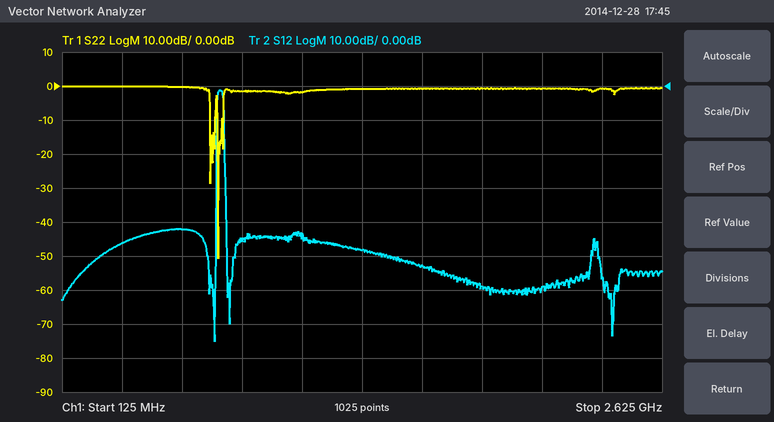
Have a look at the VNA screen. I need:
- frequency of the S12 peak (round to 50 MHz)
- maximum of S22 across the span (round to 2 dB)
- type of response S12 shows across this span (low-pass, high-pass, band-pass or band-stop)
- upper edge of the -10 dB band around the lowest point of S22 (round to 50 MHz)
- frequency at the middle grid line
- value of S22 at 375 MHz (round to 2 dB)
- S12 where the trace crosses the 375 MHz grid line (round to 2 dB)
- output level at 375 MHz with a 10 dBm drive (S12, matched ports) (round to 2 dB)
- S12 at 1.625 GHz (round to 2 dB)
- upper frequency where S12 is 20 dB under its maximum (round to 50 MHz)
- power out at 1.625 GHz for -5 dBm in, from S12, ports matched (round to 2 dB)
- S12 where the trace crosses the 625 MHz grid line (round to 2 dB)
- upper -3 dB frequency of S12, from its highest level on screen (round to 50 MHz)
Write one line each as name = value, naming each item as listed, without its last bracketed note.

frequency of the S12 peak = 800 MHz
maximum of S22 across the span = 0 dB
type of response S12 shows across this span = band-pass
upper edge of the -10 dB band around the lowest point of S22 = 800 MHz
frequency at the middle grid line = 1.375 GHz
value of S22 at 375 MHz = 0 dB
S12 where the trace crosses the 375 MHz grid line = -46 dB
output level at 375 MHz with a 10 dBm drive (S12, matched ports) = -36 dBm
S12 at 1.625 GHz = -52 dB
upper frequency where S12 is 20 dB under its maximum = 800 MHz
power out at 1.625 GHz for -5 dBm in, from S12, ports matched = -58 dBm
S12 where the trace crosses the 625 MHz grid line = -42 dB
upper -3 dB frequency of S12, from its highest level on screen = 800 MHz
